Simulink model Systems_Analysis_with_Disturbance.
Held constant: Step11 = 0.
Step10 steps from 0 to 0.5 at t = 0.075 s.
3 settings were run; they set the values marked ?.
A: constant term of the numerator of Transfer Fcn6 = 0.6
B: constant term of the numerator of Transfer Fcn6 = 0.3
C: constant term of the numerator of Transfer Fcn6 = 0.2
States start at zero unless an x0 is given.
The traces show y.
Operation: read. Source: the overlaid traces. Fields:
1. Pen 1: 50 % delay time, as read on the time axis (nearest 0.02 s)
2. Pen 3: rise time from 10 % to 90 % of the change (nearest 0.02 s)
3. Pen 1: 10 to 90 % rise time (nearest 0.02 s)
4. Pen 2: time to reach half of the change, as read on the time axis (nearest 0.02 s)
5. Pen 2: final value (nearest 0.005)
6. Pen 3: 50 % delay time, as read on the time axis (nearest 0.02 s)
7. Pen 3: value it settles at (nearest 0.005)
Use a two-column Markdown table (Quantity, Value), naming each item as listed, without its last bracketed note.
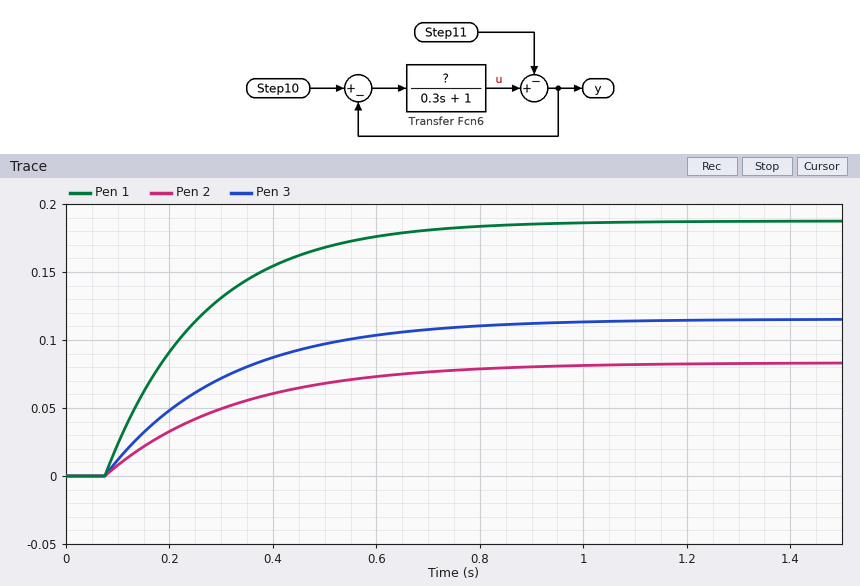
| Quantity | Value |
|---|---|
| Pen 1: 50 % delay time, as read on the time axis | 0.20 s |
| Pen 3: rise time from 10 % to 90 % of the change | 0.50 s |
| Pen 1: 10 to 90 % rise time | 0.42 s |
| Pen 2: time to reach half of the change, as read on the time axis | 0.24 s |
| Pen 2: final value | 0.085 |
| Pen 3: 50 % delay time, as read on the time axis | 0.24 s |
| Pen 3: value it settles at | 0.115 |
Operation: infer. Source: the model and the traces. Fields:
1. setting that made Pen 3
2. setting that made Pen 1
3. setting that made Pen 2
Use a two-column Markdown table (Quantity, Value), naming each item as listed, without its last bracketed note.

| Quantity | Value |
|---|---|
| setting that made Pen 3 | B |
| setting that made Pen 1 | A |
| setting that made Pen 2 | C |
